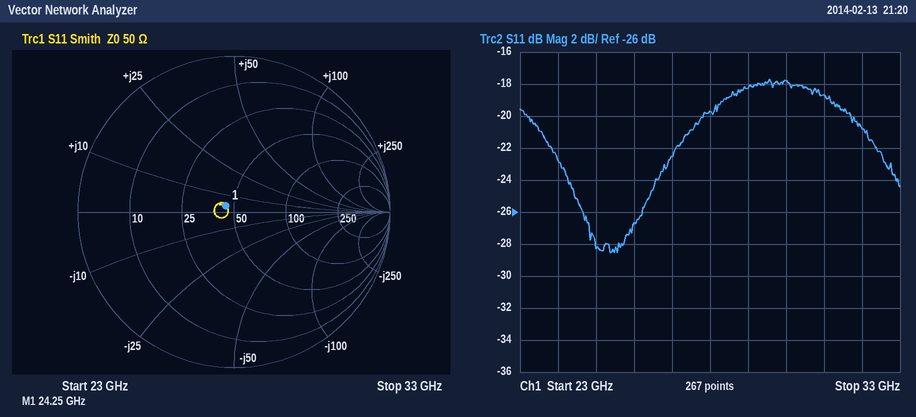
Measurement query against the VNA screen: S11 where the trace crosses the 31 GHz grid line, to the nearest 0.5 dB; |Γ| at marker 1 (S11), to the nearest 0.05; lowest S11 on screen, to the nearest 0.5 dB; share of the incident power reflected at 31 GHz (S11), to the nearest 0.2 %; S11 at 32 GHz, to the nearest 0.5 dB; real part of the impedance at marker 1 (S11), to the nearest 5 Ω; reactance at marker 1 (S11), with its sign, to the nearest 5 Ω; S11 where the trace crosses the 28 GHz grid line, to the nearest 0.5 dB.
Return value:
-18.5 dB
0.05
-28.5 dB
1.4 %
-21.0 dB
45 Ω
+5 Ω
-19.5 dB
